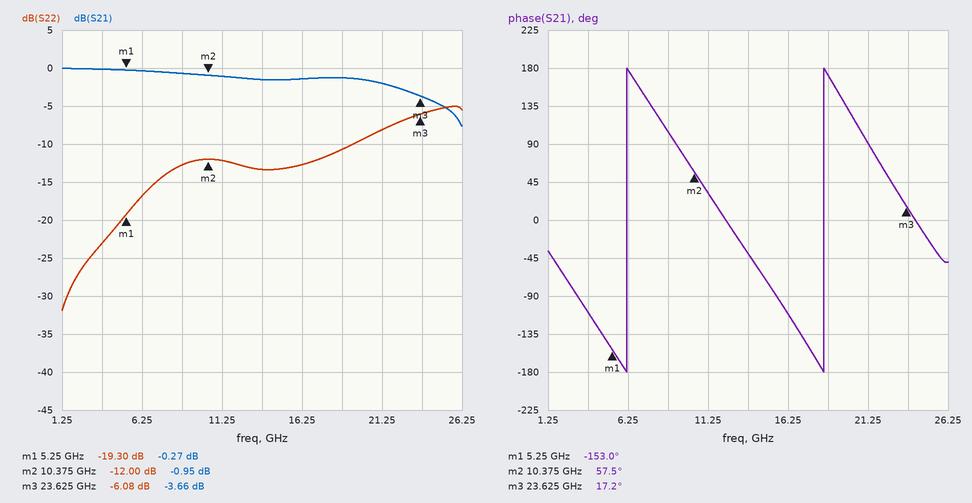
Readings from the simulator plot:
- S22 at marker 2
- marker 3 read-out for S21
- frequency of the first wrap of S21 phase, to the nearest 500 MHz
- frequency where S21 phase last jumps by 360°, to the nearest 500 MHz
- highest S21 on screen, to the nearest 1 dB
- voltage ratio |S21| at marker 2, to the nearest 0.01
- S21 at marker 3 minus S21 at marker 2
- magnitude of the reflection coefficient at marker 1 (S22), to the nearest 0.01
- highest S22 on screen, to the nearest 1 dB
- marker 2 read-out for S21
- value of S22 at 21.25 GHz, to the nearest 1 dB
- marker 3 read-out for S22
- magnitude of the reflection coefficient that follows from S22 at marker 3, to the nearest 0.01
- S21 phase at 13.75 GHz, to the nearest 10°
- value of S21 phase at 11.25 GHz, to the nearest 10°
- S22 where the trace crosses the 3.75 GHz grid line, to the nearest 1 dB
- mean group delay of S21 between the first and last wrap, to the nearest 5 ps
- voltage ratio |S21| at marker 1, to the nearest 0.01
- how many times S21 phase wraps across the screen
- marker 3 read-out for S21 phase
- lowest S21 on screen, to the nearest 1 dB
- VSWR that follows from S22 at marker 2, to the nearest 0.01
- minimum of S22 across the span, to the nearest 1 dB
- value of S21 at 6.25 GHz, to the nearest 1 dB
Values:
-12.00 dB
-3.66 dB
6.0 GHz
18.5 GHz
0 dB
0.90
-2.71 dB
0.11
-5 dB
-0.95 dB
-8 dB
-6.08 dB
0.50
-40°
30°
-23 dB
80 ps
0.97
2
17.2°
-8 dB
1.67
-32 dB
0 dB
